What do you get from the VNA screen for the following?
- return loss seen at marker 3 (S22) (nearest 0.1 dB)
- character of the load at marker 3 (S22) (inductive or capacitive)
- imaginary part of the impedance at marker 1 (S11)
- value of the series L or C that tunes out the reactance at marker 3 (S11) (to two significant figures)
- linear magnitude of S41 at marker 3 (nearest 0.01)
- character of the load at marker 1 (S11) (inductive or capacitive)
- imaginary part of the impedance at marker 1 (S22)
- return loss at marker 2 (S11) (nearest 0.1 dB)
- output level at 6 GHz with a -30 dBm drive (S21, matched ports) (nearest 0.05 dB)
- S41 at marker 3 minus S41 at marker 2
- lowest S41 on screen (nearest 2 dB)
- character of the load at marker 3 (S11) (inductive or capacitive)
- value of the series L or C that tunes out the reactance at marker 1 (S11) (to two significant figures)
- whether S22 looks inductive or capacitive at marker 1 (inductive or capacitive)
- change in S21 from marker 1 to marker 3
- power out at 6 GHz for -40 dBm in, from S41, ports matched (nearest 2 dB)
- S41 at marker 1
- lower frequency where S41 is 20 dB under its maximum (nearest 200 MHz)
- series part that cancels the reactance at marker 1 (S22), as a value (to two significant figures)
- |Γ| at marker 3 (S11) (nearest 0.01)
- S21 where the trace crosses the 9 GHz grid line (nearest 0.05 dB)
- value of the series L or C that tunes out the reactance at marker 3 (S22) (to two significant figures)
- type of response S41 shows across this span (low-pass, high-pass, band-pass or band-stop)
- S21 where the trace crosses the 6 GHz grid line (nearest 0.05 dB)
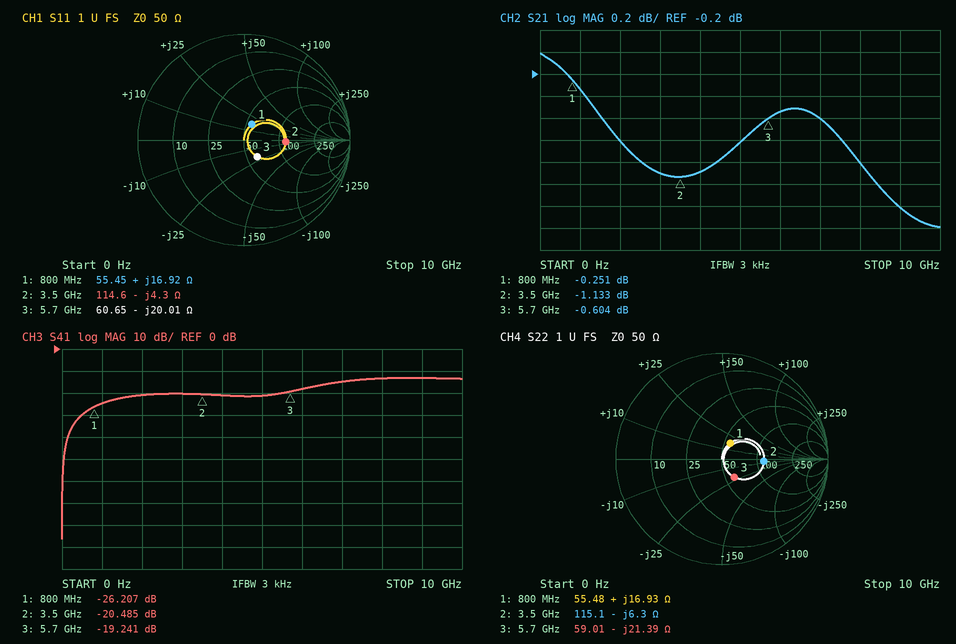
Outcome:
13.6 dB
capacitive
+16.92 Ω
560 pH
0.11
inductive
+16.93 Ω
8.1 dB
-30.55 dBm
1.244 dB
-86 dB
capacitive
12 pF
inductive
-0.353 dB
-58 dBm
-26.207 dB
400 MHz
12 pF
0.20
-1.40 dB
600 pH
high-pass
-0.55 dB
